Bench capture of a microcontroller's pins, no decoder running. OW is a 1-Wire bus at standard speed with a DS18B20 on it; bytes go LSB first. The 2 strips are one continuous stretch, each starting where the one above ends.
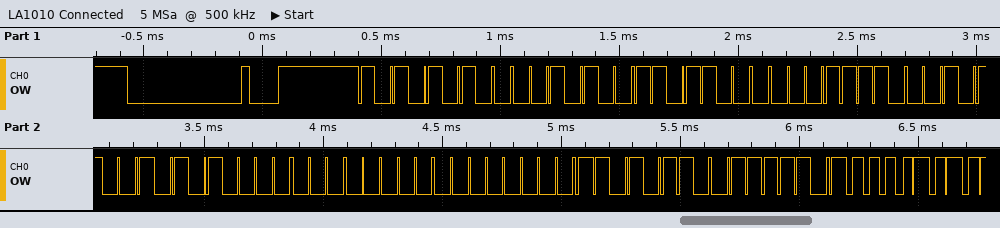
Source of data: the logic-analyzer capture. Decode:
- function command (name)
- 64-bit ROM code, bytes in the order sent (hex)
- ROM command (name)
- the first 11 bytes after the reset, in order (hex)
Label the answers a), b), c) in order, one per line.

a) Read Scratchpad
b) 28 1B 78 94 0A 00 00 6B
c) Match ROM
d) 55 28 1B 78 94 0A 00 00 6B BE 50
